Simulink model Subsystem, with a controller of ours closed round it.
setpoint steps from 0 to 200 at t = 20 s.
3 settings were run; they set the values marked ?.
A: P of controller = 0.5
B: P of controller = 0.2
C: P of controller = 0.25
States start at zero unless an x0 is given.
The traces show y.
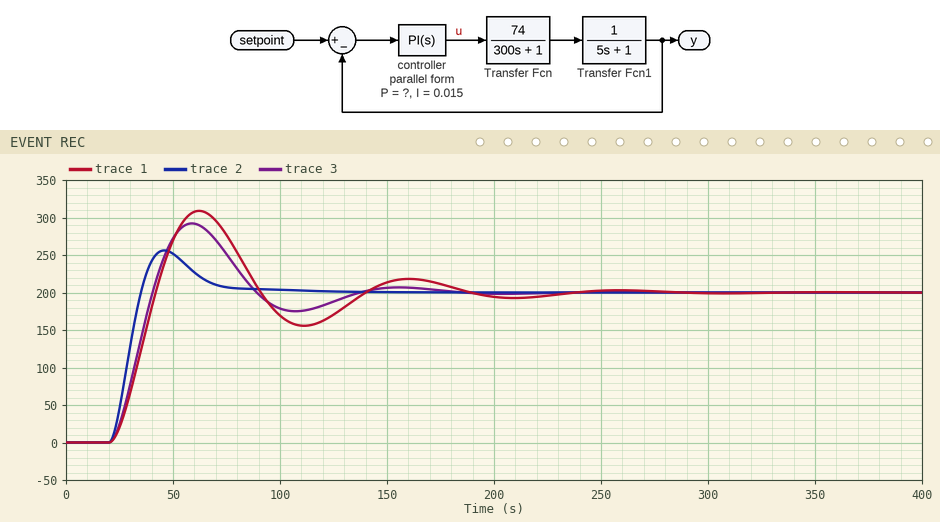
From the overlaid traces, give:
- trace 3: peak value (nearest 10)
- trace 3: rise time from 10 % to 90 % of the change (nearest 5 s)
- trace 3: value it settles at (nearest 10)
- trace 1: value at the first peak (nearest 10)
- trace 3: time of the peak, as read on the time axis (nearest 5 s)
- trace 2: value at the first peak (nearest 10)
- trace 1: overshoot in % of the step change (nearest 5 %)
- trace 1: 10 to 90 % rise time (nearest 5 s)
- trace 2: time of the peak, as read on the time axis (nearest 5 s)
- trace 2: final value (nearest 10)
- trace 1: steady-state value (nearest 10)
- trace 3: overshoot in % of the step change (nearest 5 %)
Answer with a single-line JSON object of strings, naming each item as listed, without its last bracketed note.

{"trace 3: peak value": "290", "trace 3: rise time from 10 % to 90 % of the change": "15 s", "trace 3: value it settles at": "200", "trace 1: value at the first peak": "310", "trace 3: time of the peak, as read on the time axis": "60 s", "trace 2: value at the first peak": "260", "trace 1: overshoot in % of the step change": "55 %", "trace 1: 10 to 90 % rise time": "15 s", "trace 2: time of the peak, as read on the time axis": "45 s", "trace 2: final value": "200", "trace 1: steady-state value": "200", "trace 3: overshoot in % of the step change": "45 %"}
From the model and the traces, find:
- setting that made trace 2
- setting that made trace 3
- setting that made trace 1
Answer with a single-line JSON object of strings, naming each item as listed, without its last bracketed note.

{"setting that made trace 2": "A", "setting that made trace 3": "C", "setting that made trace 1": "B"}
